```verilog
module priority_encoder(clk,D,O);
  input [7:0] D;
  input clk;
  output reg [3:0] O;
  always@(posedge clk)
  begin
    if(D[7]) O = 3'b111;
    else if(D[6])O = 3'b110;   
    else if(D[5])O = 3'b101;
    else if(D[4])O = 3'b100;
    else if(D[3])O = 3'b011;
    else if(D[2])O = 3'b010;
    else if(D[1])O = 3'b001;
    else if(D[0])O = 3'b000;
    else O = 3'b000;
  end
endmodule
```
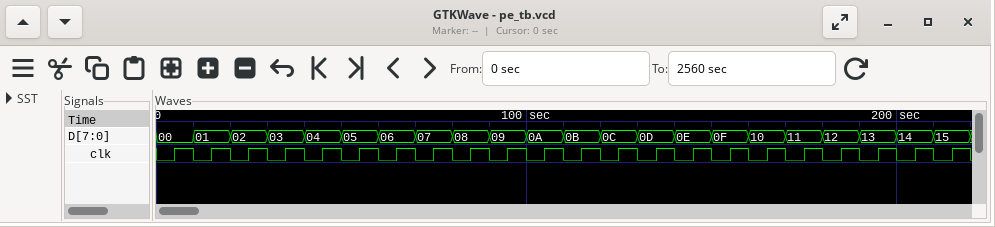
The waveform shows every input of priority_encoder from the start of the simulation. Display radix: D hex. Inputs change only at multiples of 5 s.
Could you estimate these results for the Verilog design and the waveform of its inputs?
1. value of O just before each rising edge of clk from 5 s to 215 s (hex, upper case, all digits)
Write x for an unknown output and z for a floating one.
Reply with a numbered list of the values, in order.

1. x, 0, 0, 1, 1, 2, 2, 2, 2, 3, 3, 3, 3, 3, 3, 3, 3, 4, 4, 4, 4, 4
